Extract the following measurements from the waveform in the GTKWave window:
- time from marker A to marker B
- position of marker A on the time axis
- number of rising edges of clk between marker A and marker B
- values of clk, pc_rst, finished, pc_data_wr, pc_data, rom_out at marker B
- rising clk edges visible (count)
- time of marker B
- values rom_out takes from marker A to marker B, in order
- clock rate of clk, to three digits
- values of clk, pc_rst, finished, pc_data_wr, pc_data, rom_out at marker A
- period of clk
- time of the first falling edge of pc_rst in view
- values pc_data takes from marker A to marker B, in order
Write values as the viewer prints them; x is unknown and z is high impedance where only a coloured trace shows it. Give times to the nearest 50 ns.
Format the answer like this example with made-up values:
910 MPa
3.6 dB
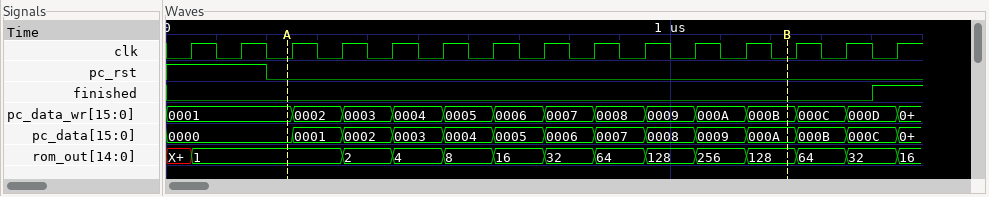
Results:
1000 ns
250 ns
10
clk=0, pc_rst=0, finished=0, pc_data_wr=000B, pc_data=000A, rom_out=128
15
1250 ns
1, 2, 4, 8, 16, 32, 64, 128, 256, 128
10.0 MHz
clk=0, pc_rst=0, finished=0, pc_data_wr=0001, pc_data=0000, rom_out=1
100 ns
200 ns
0000, 0001, 0002, 0003, 0004, 0005, 0006, 0007, 0008, 0009, 000A
